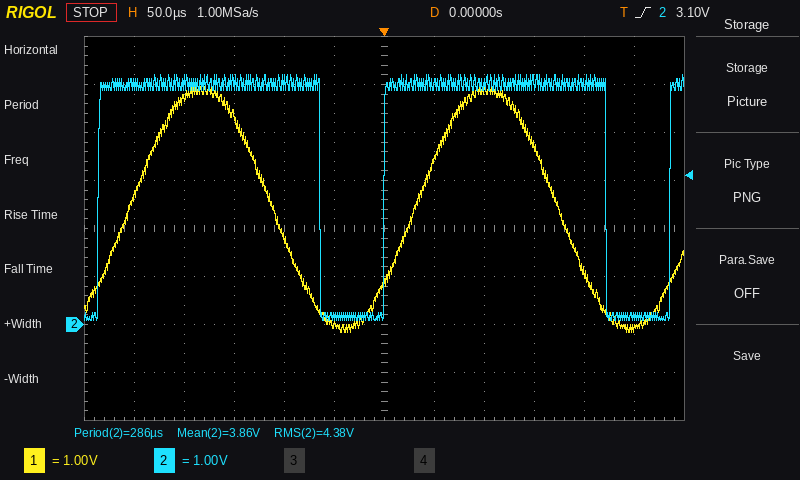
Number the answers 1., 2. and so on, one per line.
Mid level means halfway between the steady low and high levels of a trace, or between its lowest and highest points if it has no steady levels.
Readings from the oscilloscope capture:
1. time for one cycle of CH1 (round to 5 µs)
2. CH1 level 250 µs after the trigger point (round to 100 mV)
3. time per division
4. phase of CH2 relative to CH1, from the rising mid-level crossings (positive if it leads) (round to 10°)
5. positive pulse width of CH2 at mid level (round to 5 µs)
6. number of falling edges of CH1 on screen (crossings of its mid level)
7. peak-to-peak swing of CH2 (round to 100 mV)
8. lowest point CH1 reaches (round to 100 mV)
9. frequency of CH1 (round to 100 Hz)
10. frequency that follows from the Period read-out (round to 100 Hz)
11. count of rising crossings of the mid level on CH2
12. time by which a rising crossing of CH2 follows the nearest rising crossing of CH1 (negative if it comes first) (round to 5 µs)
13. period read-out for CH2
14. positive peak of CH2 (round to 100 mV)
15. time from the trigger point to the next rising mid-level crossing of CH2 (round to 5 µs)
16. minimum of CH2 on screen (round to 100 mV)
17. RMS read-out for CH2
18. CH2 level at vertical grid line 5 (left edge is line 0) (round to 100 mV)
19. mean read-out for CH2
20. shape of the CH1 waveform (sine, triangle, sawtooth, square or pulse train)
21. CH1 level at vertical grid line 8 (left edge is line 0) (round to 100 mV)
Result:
1. 285 µs
2. -100 mV
3. 50 µs
4. +40°
5. 220 µs
6. 2
7. 5.1 V
8. -200 mV
9. 3.5 kHz
10. 3.5 kHz
11. 3
12. -30 µs
13. 286 µs
14. 5.2 V
15. 285 µs
16. 100 mV
17. 4.38 V
18. 200 mV
19. 3.86 V
20. sine
21. 4.9 V
